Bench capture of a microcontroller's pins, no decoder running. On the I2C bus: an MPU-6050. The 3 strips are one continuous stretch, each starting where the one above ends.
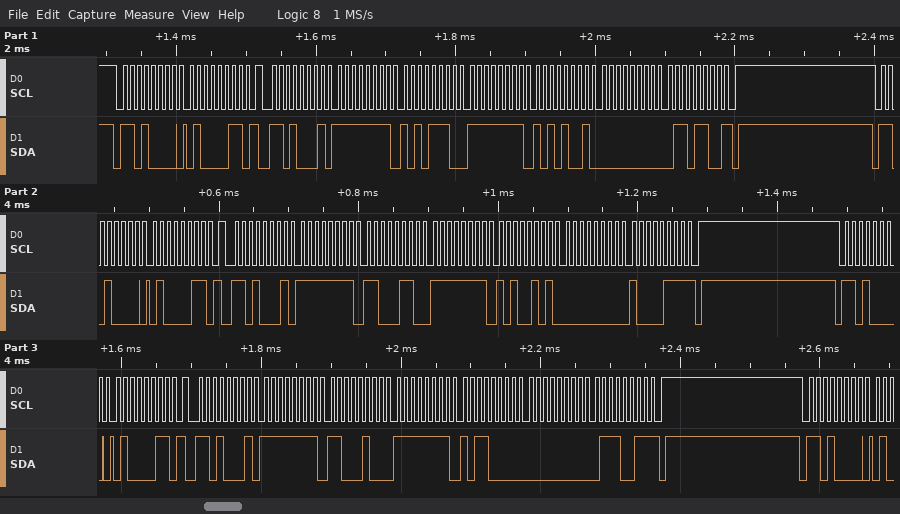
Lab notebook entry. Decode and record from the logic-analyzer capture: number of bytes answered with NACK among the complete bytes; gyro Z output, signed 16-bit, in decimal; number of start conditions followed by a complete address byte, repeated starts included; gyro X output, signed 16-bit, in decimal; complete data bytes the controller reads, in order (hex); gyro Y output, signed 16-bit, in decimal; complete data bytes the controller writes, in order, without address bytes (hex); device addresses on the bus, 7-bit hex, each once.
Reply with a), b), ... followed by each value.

a) 3
b) 108
c) 7
d) -82
e) FF AE FF A9 00 6C FF C6 FF A5 00 87 FF C4 FF B0 00 73
f) -87
g) 43 43 43
h) 0x68
